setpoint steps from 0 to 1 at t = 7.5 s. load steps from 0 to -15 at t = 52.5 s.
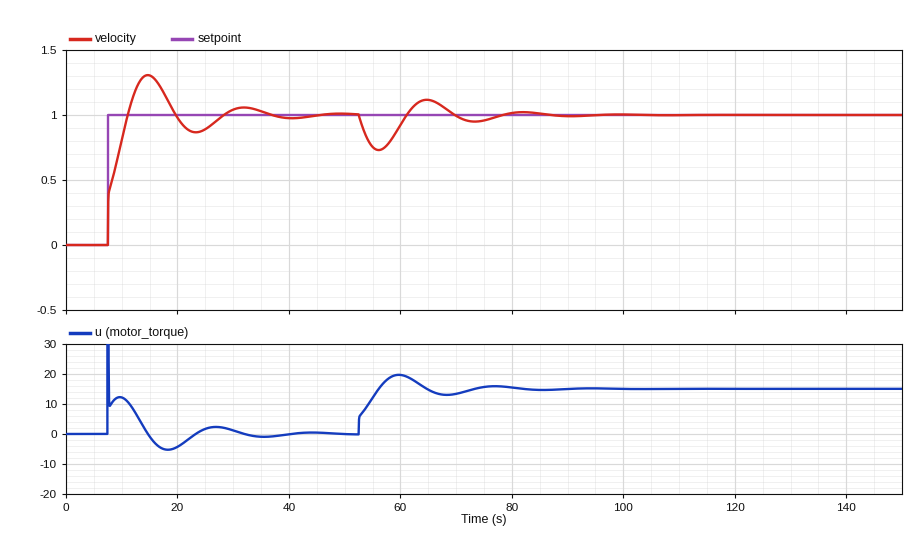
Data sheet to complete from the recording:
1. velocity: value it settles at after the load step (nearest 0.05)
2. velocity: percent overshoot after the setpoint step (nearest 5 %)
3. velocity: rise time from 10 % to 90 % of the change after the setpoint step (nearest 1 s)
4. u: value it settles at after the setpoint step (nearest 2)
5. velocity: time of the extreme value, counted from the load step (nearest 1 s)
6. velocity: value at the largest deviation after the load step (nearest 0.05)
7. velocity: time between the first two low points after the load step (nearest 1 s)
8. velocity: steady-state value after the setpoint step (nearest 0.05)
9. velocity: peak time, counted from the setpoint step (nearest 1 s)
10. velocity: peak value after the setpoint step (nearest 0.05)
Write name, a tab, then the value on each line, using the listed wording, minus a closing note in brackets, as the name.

velocity: value it settles at after the load step	1.00
velocity: percent overshoot after the setpoint step	30 %
velocity: rise time from 10 % to 90 % of the change after the setpoint step	3 s
u: value it settles at after the setpoint step	0
velocity: time of the extreme value, counted from the load step	4 s
velocity: value at the largest deviation after the load step	0.75
velocity: time between the first two low points after the load step	17 s
velocity: steady-state value after the setpoint step	1.00
velocity: peak time, counted from the setpoint step	7 s
velocity: peak value after the setpoint step	1.30
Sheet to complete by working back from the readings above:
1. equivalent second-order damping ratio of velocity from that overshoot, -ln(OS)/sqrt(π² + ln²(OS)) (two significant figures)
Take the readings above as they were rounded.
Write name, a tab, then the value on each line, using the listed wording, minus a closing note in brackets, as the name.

equivalent second-order damping ratio of velocity from that overshoot, -ln(OS)/sqrt(π² + ln²(OS))	0.36
